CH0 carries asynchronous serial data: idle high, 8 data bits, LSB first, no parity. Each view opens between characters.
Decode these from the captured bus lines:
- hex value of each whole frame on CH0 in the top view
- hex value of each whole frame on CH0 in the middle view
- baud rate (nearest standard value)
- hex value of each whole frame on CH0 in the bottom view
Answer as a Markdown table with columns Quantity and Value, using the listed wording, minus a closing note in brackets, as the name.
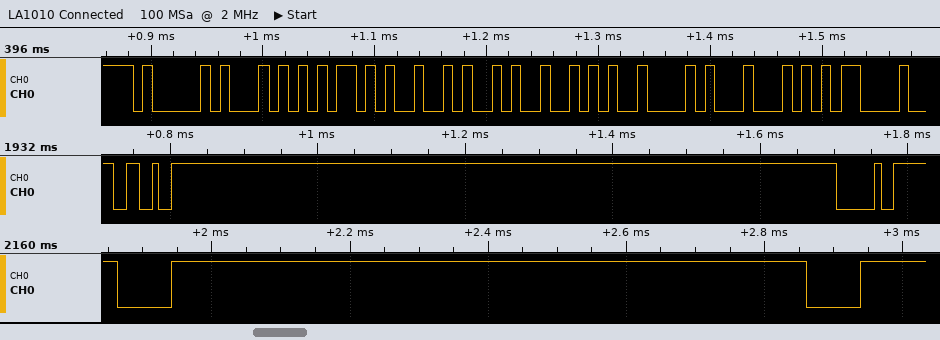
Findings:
| Quantity | Value |
|---|---|
| hex value of each whole frame on CH0 in the top view | 41, 54, 2B, 4A, 52, 42, 44, 0D |
| hex value of each whole frame on CH0 in the middle view | 26, 20 |
| baud rate | 115200 baud |
| hex value of each whole frame on CH0 in the bottom view | 00, 00 |
